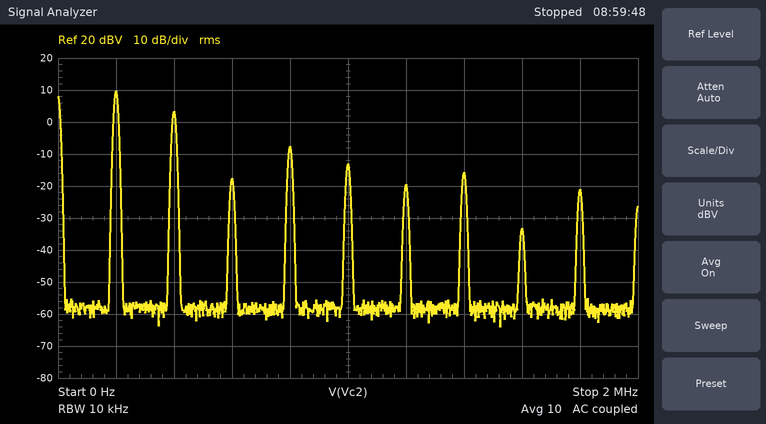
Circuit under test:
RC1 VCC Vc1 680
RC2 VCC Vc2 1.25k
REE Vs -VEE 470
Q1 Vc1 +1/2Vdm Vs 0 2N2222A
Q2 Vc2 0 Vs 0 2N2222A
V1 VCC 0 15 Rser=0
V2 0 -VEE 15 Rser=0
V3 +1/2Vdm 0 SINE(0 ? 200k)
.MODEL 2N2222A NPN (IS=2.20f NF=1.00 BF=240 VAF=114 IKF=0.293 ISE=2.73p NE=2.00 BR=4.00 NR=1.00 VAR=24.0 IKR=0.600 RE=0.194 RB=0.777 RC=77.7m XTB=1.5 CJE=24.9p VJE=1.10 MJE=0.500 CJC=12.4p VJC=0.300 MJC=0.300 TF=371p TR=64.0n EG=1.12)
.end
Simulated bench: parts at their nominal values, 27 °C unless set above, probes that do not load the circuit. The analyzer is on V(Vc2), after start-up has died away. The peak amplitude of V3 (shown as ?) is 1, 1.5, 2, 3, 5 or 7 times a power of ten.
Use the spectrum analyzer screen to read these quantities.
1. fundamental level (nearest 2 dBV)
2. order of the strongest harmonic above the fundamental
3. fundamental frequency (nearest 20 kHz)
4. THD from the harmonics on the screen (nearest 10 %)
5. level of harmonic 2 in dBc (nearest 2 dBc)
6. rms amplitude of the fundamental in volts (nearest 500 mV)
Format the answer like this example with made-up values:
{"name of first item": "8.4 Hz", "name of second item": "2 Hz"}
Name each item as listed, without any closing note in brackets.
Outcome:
{"fundamental level": "10 dBV", "order of the strongest harmonic above the fundamental": "2", "fundamental frequency": "200 kHz", "THD from the harmonics on the screen": "50 %", "level of harmonic 2 in dBc": "-6 dBc", "rms amplitude of the fundamental in volts": "3.0 V"}
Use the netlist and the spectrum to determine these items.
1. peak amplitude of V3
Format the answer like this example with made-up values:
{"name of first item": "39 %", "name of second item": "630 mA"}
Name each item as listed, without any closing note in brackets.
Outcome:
{"peak amplitude of V3": "50 mV"}
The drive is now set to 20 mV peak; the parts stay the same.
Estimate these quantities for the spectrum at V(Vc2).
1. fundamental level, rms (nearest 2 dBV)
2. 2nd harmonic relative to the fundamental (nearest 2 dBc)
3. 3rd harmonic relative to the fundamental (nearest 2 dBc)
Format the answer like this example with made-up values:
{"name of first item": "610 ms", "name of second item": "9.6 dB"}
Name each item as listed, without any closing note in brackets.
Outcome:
{"fundamental level, rms": "-2 dBV", "2nd harmonic relative to the fundamental": "-4 dBc", "3rd harmonic relative to the fundamental": "-10 dBc"}
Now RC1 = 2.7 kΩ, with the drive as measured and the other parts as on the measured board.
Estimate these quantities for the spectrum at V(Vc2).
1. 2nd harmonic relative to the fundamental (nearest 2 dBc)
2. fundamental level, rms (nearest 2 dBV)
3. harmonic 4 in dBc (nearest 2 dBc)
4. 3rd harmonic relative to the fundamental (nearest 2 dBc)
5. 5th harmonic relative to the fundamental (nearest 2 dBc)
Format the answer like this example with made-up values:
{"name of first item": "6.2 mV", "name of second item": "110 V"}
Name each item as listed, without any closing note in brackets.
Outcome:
{"2nd harmonic relative to the fundamental": "-10 dBc", "fundamental level, rms": "-30 dBV", "harmonic 4 in dBc": "-22 dBc", "3rd harmonic relative to the fundamental": "-16 dBc", "5th harmonic relative to the fundamental": "-26 dBc"}
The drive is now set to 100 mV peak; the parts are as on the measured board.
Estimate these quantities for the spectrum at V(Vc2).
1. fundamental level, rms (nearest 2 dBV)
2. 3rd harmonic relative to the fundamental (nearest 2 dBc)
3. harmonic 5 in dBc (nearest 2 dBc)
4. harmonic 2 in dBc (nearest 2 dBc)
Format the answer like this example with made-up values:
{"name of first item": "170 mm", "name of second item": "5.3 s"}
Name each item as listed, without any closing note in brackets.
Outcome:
{"fundamental level, rms": "14 dBV", "3rd harmonic relative to the fundamental": "-24 dBc", "harmonic 5 in dBc": "-30 dBc", "harmonic 2 in dBc": "-8 dBc"}
